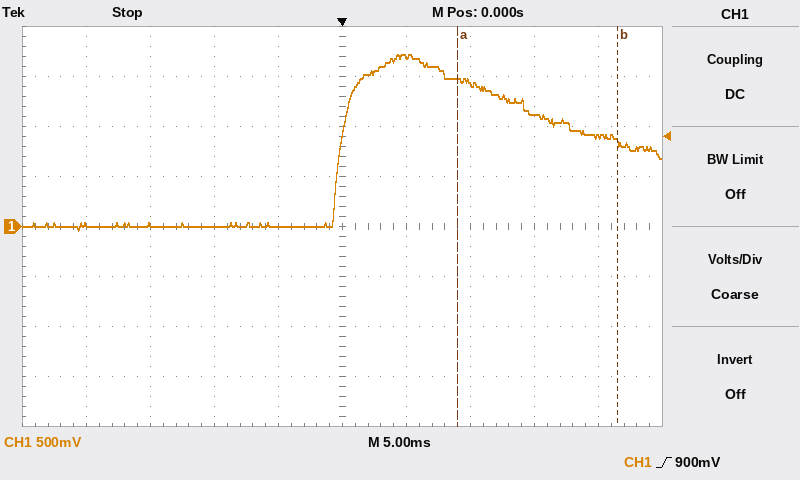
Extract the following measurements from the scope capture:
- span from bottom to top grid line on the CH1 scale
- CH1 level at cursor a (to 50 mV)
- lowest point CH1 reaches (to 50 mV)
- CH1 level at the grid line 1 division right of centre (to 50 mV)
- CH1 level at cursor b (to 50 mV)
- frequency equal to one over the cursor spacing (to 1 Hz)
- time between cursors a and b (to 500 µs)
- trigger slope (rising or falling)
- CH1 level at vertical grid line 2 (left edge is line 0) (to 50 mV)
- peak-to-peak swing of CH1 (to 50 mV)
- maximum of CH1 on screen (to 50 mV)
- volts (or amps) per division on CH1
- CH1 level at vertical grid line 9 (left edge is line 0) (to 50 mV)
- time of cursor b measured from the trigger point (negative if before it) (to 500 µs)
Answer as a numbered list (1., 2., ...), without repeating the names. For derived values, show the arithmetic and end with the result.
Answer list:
1. 4 V
2. 1.45 V
3. -50 mV
4. 1.70 V
5. 850 mV
6. 1 / 12.5 ms ≈ 80 Hz
7. 12.5 ms
8. rising
9. 0 mV
10. 1.70 V − (-50 mV) = 1.75 V
11. 1.70 V
12. 500 mV
13. 900 mV
14. +21.5 ms
